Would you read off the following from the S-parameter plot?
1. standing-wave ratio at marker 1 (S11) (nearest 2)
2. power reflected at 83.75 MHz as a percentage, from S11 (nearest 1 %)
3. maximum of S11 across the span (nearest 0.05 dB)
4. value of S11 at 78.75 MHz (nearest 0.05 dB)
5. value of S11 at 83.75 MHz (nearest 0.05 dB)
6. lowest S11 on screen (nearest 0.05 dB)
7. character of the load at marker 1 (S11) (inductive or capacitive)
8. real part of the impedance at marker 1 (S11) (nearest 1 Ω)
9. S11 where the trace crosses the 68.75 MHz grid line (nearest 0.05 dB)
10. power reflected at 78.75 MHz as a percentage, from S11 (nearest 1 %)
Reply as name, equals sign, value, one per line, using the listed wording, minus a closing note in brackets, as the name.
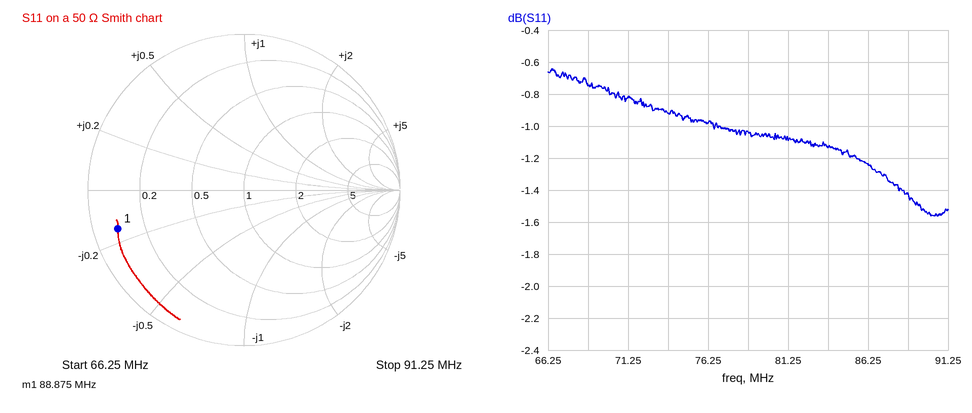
standing-wave ratio at marker 1 (S11) = 12
power reflected at 83.75 MHz as a percentage, from S11 = 77 %
maximum of S11 across the span = -0.65 dB
value of S11 at 78.75 MHz = -1.05 dB
value of S11 at 83.75 MHz = -1.15 dB
lowest S11 on screen = -1.55 dB
character of the load at marker 1 (S11) = capacitive
real part of the impedance at marker 1 (S11) = 4 Ω
S11 where the trace crosses the 68.75 MHz grid line = -0.75 dB
power reflected at 78.75 MHz as a percentage, from S11 = 79 %
